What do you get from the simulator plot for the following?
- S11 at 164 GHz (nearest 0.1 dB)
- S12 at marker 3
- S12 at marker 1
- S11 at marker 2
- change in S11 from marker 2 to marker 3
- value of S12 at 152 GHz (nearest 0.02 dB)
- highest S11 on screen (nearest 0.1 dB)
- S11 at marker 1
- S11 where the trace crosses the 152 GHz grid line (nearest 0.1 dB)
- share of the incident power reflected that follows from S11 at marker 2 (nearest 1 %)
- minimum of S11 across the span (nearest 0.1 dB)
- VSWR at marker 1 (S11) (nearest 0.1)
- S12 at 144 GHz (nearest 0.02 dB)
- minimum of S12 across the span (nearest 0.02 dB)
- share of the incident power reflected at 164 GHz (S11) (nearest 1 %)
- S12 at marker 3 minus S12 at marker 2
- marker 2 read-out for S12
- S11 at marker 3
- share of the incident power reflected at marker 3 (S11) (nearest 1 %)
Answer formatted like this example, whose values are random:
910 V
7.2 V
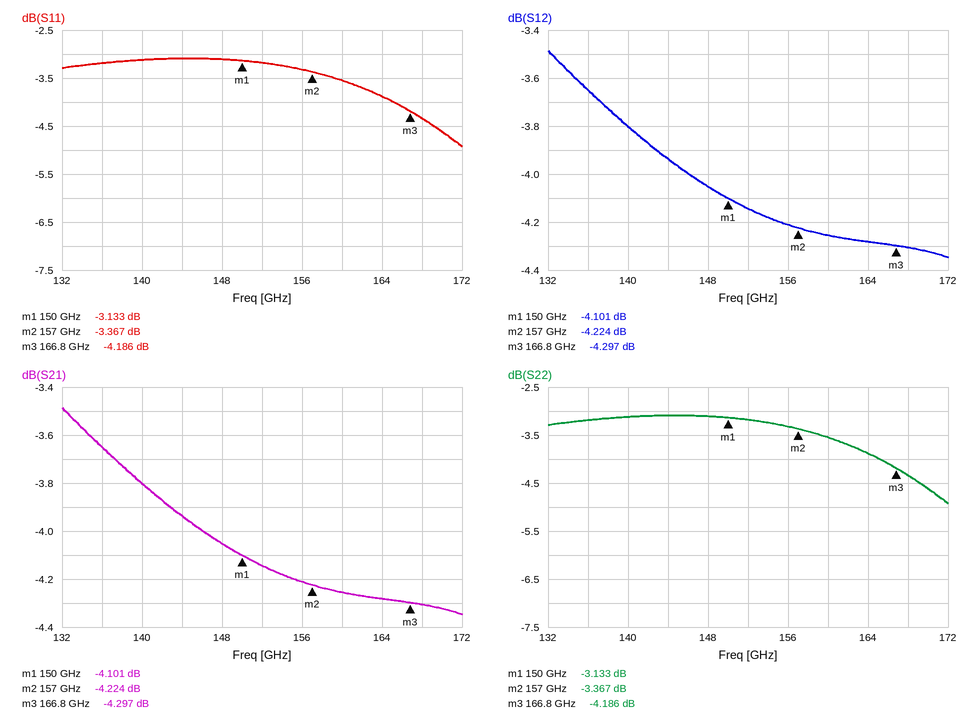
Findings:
-3.9 dB
-4.297 dB
-4.101 dB
-3.367 dB
-0.819 dB
-4.14 dB
-3.1 dB
-3.133 dB
-3.2 dB
46 %
-4.9 dB
5.6
-3.94 dB
-4.34 dB
41 %
-0.073 dB
-4.224 dB
-4.186 dB
38 %
